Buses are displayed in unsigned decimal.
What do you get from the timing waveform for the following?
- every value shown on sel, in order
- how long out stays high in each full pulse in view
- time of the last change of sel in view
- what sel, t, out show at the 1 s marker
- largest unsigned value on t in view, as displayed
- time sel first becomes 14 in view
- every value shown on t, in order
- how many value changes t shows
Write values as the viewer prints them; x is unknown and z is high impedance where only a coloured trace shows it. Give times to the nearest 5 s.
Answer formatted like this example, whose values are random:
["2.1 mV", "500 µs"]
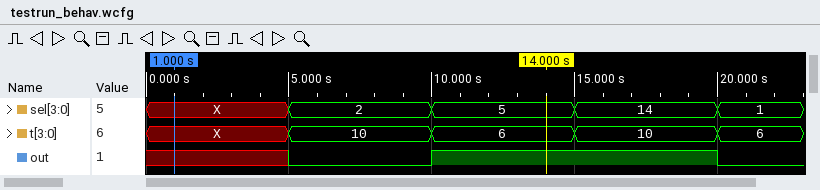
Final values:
["X, 2, 5, 14, 1", "10 s", "20 s", "sel=X, t=X, out=x", "10", "15 s", "X, 10, 6, 10, 6", "4"]
